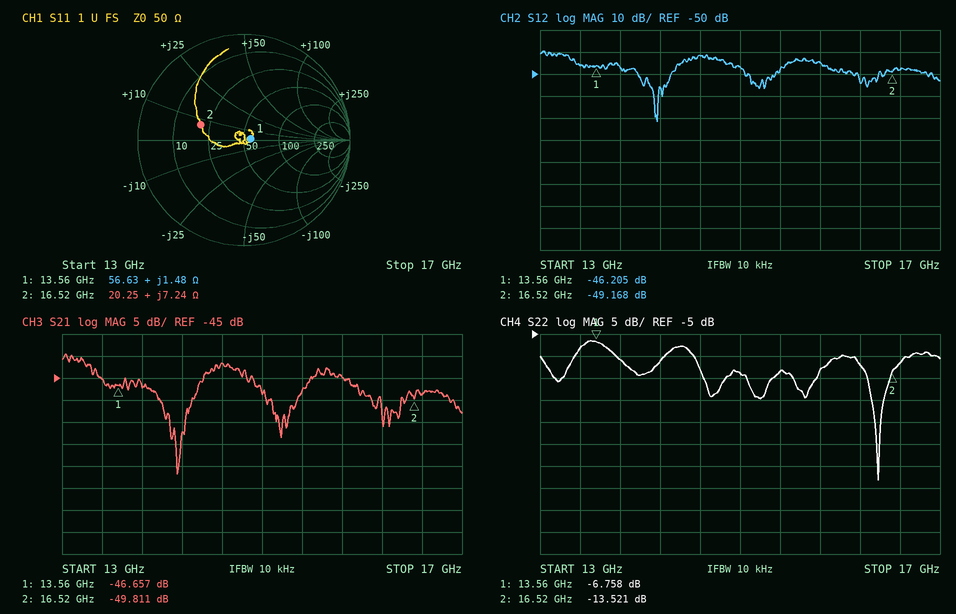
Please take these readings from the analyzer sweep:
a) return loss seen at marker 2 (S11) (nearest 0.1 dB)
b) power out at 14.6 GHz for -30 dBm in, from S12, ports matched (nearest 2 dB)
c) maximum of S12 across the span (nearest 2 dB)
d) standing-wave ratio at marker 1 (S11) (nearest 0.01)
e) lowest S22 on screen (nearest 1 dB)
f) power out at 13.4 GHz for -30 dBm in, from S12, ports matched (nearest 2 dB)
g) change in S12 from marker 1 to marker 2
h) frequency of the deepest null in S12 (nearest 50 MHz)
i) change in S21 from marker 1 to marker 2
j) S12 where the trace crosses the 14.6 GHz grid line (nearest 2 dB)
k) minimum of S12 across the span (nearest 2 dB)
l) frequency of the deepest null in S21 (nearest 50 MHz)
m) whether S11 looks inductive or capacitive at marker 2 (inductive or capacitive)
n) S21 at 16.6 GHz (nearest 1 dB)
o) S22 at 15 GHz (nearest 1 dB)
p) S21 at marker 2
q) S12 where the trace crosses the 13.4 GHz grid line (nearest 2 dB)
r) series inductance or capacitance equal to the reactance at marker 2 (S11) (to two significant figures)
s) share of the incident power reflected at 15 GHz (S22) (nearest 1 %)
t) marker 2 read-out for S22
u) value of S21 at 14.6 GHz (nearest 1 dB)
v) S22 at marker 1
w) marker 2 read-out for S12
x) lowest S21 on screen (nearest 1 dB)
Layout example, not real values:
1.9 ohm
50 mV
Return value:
7.3 dB
-72 dBm
-40 dB
1.14
-38 dB
-76 dBm
-2.963 dB
14.15 GHz
-3.154 dB
-42 dB
-72 dB
14.15 GHz
inductive
-49 dB
-14 dB
-49.811 dB
-46 dB
70 pH
4 %
-13.521 dB
-42 dB
-6.758 dB
-49.168 dB
-67 dB
